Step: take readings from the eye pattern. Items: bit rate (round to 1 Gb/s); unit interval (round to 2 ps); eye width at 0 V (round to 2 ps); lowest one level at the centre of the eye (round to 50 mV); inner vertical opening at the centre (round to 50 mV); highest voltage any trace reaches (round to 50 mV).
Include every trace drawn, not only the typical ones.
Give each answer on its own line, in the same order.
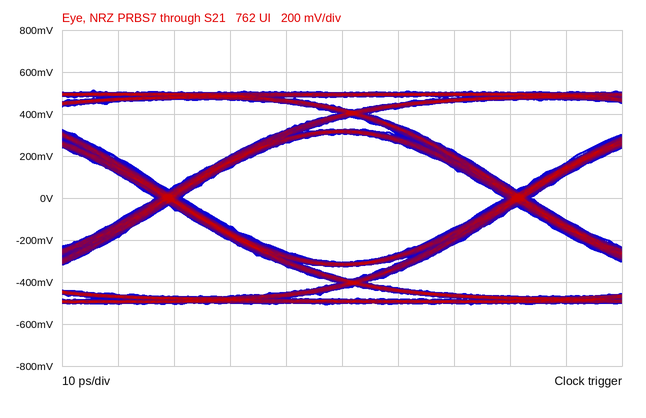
16 Gb/s
62 ps
58 ps
300 mV
600 mV
500 mV
